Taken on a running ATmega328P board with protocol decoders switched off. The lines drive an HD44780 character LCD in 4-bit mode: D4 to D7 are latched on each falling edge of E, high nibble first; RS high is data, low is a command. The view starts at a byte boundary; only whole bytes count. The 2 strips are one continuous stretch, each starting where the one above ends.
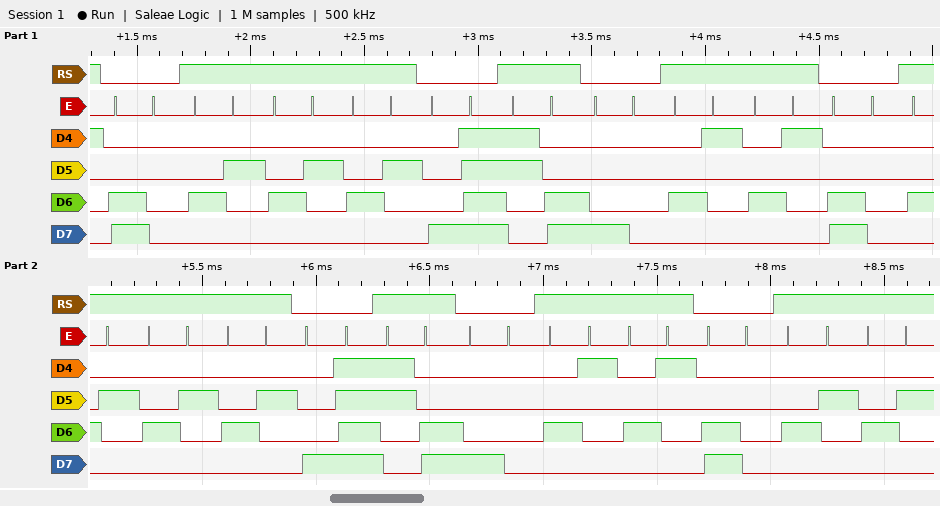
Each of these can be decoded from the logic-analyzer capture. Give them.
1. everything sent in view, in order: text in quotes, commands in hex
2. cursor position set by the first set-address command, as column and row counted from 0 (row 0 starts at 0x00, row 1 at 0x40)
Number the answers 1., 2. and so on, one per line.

1. 0xC0 "BBB" 0x8F "<" 0x80 "AA" 0xC0 "BBB" 0x8F "<" 0x80 "AA" 0xC0 "BB"
2. column 0, row 1
